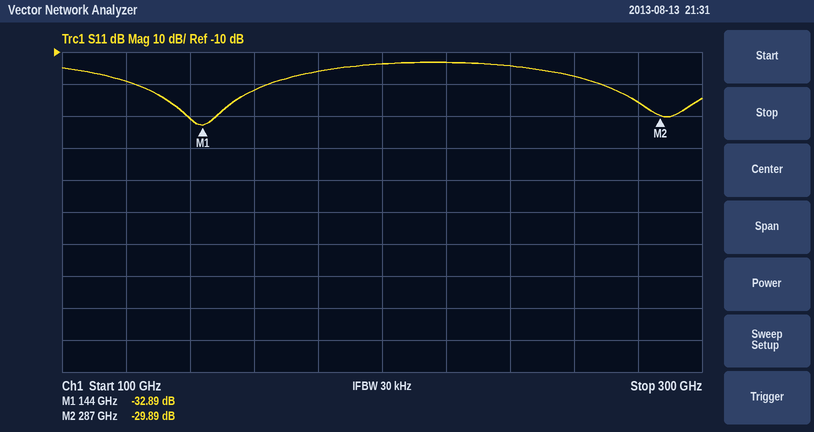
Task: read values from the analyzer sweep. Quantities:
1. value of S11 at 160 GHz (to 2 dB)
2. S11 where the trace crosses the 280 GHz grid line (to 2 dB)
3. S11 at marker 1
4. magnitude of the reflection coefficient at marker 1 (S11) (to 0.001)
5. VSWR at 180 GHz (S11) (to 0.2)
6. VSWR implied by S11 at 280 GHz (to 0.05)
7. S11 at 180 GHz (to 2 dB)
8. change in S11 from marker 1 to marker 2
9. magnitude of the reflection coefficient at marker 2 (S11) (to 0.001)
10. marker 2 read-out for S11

-22 dB
-26 dB
-32.89 dB
0.023
1.4
1.10
-16 dB
3.00 dB
0.032
-29.89 dB
